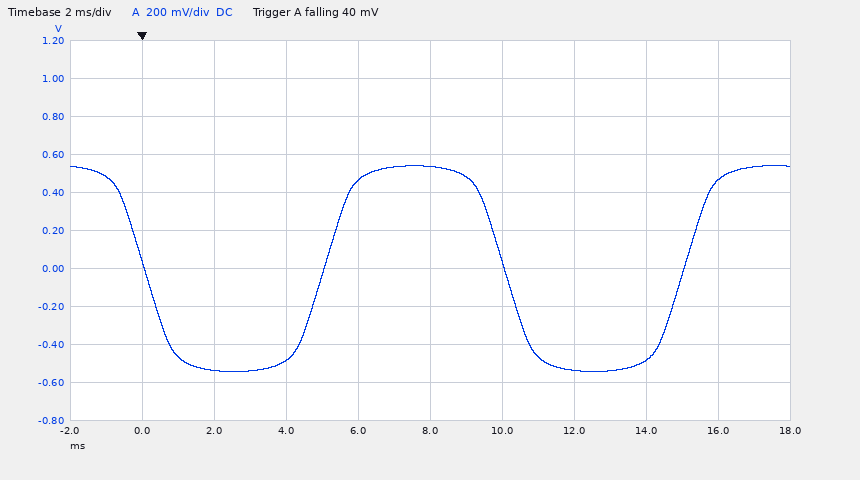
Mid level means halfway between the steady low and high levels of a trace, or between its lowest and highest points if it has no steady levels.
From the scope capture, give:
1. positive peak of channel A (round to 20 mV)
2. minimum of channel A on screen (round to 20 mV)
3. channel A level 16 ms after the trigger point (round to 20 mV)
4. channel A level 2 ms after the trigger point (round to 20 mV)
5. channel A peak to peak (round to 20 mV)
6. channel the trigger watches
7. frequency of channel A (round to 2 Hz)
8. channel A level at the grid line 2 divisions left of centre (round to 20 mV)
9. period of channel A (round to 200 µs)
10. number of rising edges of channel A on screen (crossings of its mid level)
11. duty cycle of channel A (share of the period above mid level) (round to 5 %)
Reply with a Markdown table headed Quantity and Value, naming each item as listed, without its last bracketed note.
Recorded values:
| Quantity | Value |
|---|---|
| positive peak of channel A | 540 mV |
| minimum of channel A on screen | -540 mV |
| channel A level 16 ms after the trigger point | 460 mV |
| channel A level 2 ms after the trigger point | -540 mV |
| channel A peak to peak | 1.08 V |
| channel the trigger watches | channel A |
| frequency of channel A | 100 Hz |
| channel A level at the grid line 2 divisions left of centre | -480 mV |
| period of channel A | 10.0 ms |
| number of rising edges of channel A on screen | 2 |
| duty cycle of channel A (share of the period above mid level) | 50 % |
